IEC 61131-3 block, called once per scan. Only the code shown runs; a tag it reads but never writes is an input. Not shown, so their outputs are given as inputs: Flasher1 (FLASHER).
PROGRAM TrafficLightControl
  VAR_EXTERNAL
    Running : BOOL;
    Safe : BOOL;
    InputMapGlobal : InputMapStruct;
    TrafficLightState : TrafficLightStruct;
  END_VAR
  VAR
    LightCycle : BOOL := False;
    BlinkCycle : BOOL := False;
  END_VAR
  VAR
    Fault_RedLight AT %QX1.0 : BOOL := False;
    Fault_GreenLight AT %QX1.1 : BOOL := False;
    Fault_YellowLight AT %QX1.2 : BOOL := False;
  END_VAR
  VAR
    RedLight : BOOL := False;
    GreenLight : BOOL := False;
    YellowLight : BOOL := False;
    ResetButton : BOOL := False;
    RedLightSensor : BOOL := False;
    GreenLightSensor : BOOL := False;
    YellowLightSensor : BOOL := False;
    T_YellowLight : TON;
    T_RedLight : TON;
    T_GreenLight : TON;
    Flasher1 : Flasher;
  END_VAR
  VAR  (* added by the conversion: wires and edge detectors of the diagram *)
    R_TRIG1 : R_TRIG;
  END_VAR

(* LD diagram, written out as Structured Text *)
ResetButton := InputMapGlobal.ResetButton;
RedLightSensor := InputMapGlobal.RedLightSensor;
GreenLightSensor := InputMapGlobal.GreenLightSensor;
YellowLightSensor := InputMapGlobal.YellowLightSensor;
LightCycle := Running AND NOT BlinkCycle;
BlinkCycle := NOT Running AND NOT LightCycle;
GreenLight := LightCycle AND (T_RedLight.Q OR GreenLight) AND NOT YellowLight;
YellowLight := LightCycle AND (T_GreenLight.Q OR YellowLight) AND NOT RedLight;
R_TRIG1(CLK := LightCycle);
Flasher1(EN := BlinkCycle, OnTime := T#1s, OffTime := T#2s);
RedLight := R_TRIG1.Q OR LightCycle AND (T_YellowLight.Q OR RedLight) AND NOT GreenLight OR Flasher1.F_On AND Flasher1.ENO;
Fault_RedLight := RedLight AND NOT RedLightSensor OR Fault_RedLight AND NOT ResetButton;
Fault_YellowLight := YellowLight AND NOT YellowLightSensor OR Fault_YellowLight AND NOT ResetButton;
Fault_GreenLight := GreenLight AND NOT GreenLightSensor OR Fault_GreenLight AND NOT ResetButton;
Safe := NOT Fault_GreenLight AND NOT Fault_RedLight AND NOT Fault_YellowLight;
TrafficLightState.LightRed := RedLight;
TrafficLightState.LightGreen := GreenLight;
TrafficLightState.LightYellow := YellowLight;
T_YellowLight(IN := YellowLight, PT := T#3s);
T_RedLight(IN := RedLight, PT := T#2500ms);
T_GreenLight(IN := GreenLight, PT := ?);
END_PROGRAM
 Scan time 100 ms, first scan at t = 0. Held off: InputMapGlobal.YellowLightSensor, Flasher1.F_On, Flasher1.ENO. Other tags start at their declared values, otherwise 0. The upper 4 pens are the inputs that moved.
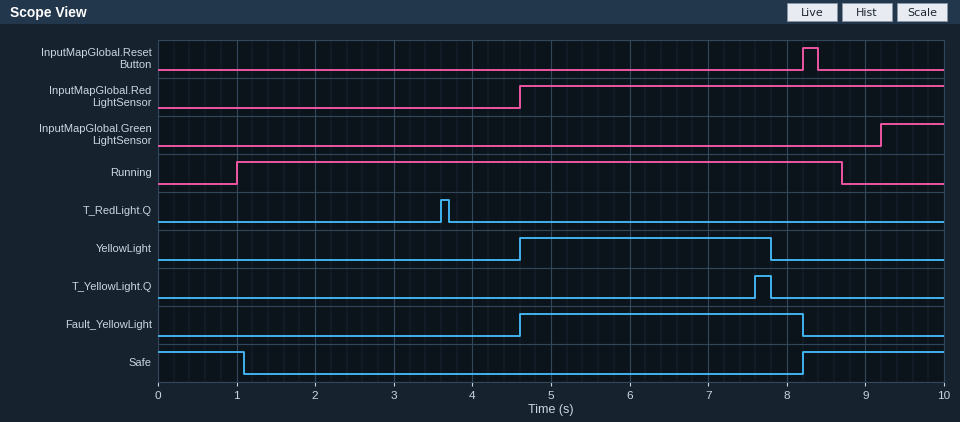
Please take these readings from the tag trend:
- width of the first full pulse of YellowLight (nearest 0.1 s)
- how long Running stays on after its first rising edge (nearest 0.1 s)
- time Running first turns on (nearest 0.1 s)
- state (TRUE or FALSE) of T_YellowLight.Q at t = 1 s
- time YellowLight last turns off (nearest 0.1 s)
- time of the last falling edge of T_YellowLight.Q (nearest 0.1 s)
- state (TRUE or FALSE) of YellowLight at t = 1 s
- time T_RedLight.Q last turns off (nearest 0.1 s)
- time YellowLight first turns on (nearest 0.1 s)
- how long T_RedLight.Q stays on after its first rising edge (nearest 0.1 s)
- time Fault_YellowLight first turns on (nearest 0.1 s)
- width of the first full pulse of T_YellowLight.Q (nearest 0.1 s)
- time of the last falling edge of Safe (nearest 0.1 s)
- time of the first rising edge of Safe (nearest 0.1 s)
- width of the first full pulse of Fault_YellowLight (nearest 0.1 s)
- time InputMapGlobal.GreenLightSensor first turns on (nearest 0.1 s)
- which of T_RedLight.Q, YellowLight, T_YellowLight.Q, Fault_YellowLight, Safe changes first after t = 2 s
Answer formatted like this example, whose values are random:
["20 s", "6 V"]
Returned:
["3.2 s", "7.7 s", "1.0 s", "FALSE", "7.8 s", "7.8 s", "FALSE", "3.7 s", "4.6 s", "0.1 s", "4.6 s", "0.2 s", "1.1 s", "8.2 s", "3.6 s", "9.2 s", "T_RedLight.Q"]
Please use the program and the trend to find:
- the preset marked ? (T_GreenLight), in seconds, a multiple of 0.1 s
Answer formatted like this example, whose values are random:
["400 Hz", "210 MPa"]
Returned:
["0.8 s"]
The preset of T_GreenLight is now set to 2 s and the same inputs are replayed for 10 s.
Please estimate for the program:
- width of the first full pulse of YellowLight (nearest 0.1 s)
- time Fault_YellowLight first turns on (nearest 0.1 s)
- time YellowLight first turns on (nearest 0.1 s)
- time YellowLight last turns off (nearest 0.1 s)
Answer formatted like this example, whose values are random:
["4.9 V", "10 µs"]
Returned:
["2.9 s", "5.8 s", "5.8 s", "8.7 s"]
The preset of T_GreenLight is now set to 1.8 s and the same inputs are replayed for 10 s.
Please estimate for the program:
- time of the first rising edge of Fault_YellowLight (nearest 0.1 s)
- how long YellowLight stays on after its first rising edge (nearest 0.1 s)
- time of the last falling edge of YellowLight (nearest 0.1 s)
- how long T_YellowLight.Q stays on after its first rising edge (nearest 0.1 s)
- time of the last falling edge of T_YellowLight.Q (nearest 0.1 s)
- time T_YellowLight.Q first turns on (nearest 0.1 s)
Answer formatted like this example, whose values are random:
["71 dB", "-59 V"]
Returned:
["5.6 s", "3.1 s", "8.7 s", "0.1 s", "8.7 s", "8.6 s"]
